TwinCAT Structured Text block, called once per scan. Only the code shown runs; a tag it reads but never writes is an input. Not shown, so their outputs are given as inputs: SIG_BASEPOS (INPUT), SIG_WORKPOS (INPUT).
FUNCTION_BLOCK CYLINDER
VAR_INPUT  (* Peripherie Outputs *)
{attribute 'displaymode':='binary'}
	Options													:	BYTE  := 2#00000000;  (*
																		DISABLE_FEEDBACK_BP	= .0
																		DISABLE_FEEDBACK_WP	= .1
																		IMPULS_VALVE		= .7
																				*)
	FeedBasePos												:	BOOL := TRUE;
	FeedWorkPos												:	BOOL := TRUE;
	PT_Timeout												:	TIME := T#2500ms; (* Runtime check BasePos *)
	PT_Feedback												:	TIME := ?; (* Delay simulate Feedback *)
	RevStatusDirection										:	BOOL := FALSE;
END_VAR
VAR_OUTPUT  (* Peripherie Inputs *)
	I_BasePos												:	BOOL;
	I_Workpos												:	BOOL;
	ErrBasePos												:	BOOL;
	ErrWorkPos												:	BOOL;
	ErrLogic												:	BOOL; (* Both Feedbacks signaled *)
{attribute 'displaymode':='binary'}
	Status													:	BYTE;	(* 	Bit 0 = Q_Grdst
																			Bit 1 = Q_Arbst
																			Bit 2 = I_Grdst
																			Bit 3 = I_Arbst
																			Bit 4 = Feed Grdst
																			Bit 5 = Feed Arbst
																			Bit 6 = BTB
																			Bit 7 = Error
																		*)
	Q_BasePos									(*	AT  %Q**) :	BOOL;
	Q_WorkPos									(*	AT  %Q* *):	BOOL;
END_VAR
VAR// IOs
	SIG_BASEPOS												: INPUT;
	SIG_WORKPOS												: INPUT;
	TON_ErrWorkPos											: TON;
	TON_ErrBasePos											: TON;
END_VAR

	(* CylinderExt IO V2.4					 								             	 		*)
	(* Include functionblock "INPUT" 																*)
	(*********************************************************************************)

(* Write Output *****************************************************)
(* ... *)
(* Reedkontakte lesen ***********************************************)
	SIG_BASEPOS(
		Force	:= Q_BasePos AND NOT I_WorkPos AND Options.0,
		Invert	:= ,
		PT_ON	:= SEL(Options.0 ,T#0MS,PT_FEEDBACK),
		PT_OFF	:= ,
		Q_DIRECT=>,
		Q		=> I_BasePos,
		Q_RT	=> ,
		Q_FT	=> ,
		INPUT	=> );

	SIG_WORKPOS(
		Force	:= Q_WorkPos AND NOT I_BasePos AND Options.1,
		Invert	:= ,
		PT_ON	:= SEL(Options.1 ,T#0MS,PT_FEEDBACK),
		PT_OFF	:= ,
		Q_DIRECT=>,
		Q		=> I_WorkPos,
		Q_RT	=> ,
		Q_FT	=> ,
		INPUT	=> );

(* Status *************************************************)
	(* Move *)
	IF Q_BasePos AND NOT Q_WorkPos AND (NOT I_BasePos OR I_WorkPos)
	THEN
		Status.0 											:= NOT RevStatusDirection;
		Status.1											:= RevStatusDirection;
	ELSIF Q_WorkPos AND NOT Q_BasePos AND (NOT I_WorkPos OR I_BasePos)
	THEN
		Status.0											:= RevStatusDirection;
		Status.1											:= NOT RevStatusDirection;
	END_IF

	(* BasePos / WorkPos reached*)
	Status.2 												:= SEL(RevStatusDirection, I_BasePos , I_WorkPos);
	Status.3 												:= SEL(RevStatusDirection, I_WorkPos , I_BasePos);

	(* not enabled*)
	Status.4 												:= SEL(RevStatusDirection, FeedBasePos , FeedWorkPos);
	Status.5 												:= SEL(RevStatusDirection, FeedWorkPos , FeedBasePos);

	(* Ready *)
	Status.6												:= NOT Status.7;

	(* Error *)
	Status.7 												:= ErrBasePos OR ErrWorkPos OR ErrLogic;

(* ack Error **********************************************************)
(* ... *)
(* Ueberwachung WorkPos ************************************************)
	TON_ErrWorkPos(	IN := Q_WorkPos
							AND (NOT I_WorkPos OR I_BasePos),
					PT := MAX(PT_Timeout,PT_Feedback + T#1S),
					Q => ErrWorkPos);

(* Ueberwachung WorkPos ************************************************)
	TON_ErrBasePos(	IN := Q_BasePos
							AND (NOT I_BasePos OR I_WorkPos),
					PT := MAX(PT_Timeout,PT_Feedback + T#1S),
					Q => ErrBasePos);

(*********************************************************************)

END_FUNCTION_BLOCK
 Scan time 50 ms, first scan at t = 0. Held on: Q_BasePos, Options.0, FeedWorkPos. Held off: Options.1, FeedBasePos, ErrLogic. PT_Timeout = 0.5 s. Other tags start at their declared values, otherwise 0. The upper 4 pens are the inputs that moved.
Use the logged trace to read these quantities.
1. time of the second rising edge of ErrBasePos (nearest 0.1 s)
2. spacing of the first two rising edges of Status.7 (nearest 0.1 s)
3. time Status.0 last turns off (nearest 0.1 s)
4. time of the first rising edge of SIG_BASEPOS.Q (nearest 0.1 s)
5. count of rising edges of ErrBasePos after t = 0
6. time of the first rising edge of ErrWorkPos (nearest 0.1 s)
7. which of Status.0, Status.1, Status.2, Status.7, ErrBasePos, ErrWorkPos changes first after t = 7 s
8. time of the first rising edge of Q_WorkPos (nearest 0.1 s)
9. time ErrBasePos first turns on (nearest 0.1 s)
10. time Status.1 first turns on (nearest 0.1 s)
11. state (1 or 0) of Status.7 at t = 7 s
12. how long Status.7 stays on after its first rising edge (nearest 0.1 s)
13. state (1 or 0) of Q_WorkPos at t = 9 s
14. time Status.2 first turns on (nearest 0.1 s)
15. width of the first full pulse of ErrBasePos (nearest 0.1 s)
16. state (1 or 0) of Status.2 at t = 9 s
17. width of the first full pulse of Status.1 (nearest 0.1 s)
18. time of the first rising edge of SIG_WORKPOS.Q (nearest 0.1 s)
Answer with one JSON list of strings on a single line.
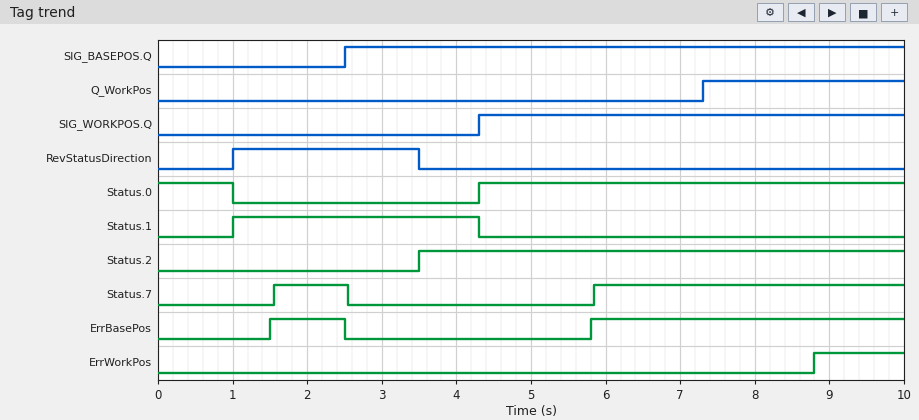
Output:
["5.8 s", "4.3 s", "1.0 s", "2.5 s", "2", "8.8 s", "ErrWorkPos", "7.3 s", "1.5 s", "1.0 s", "1", "1.0 s", "1", "3.5 s", "1.0 s", "1", "3.3 s", "4.3 s"]
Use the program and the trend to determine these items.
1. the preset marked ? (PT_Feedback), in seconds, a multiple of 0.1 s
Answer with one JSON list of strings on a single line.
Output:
["0.5 s"]
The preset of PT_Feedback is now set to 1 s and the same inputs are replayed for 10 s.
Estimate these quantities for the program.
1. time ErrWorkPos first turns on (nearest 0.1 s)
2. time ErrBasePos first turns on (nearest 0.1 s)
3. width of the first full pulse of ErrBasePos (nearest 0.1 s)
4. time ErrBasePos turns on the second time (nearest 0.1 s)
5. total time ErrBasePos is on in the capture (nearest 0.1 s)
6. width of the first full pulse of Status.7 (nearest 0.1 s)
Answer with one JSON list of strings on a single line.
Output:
["9.3 s", "2.0 s", "0.5 s", "6.3 s", "4.2 s", "0.5 s"]
